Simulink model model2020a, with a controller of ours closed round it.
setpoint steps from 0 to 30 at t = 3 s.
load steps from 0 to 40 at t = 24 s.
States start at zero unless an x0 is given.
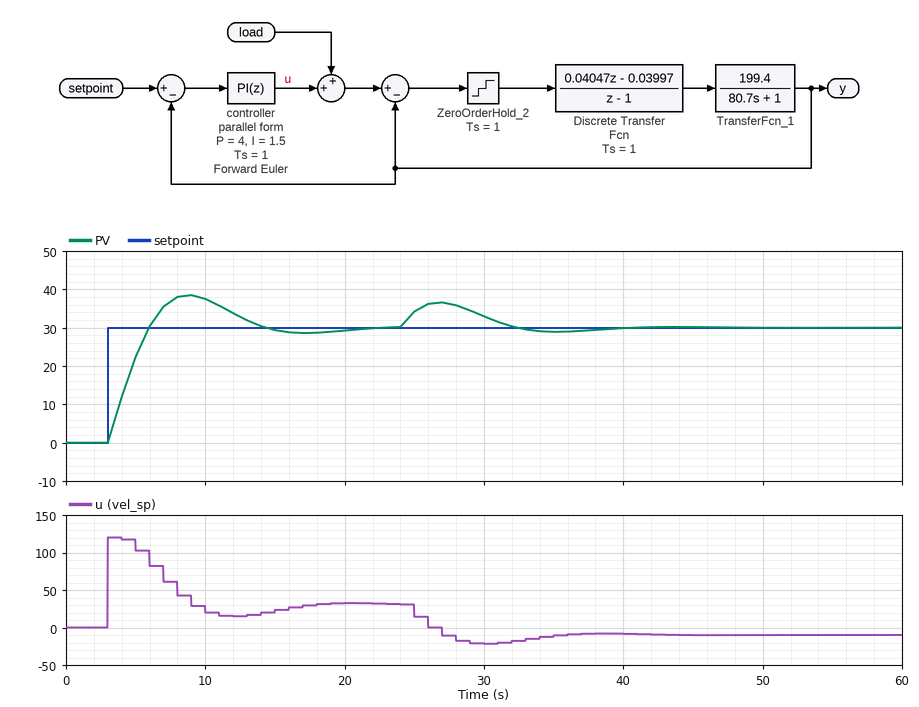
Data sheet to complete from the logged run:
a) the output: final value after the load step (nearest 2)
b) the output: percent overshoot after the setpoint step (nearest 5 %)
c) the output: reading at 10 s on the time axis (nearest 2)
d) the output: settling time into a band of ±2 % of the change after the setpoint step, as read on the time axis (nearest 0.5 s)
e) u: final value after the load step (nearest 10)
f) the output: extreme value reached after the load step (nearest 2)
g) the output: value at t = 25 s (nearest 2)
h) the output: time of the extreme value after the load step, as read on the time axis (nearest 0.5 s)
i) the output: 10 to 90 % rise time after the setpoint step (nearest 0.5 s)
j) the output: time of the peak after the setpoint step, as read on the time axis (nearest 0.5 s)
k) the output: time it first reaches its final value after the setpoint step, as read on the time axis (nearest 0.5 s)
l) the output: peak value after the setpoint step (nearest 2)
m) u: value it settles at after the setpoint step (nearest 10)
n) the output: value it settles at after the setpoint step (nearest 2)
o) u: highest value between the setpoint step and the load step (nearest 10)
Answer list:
30
30 %
38
20.5 s
-10
36
34
27.0 s
2.5 s
9.0 s
6.0 s
38
30
30
120
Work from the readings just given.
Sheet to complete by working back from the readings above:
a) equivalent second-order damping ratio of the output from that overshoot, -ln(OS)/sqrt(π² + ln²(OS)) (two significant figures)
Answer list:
0.36
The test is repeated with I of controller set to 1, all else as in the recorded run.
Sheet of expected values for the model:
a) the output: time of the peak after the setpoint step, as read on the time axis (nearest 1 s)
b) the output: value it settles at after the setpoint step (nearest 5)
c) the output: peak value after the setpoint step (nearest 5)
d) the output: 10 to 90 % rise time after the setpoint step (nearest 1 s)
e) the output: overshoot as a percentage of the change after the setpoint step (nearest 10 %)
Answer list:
10 s
30
35
3 s
20 %
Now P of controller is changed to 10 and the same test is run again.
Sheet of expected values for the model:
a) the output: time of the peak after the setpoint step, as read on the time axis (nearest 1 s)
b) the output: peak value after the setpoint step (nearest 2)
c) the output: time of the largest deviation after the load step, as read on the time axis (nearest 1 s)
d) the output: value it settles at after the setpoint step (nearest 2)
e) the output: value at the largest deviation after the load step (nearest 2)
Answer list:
5 s
32
25 s
30
34
